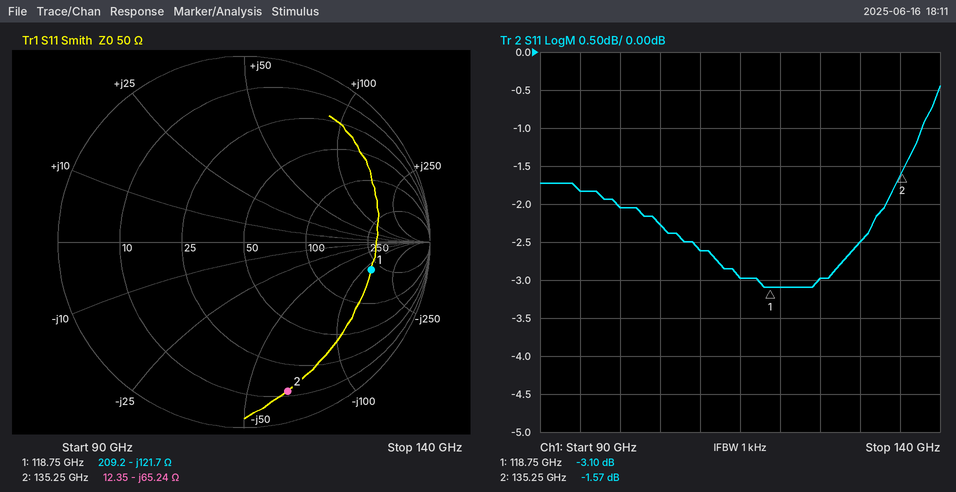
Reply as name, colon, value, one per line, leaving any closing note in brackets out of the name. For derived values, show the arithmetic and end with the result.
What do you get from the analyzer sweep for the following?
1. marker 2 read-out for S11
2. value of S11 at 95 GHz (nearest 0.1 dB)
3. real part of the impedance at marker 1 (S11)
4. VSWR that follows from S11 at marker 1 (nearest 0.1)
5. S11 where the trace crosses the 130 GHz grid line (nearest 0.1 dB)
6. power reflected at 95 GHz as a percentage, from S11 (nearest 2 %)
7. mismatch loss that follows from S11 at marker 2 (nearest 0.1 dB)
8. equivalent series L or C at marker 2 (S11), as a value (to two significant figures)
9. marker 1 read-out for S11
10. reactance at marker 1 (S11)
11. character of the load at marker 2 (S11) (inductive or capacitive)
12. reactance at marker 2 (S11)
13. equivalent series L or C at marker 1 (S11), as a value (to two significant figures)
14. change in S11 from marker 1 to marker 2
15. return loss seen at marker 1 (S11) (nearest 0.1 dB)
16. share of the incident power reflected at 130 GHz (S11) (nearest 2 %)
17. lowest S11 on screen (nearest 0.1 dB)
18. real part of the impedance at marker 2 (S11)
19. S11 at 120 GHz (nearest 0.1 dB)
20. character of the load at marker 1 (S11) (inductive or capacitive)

marker 2 read-out for S11: -1.57 dB
value of S11 at 95 GHz: -1.8 dB
real part of the impedance at marker 1: 209.2 Ω
VSWR that follows from S11 at marker 1: (1 + 0.6998)/(1 − 0.6998) ≈ 5.7
S11 where the trace crosses the 130 GHz grid line: -2.5 dB
power reflected at 95 GHz as a percentage, from S11: 10^(-1.8/10) ≈ 66 %
mismatch loss that follows from S11 at marker 2: −10 log10(1 − 10^(-1.57/10)) ≈ 5.2 dB
equivalent series L or C at marker 2 (S11), as a value: C = 1/(2π × 135.25 GHz × 65.24 Ω) ≈ 18 fF
marker 1 read-out for S11: -3.10 dB
reactance at marker 1: -121.7 Ω
character of the load at marker 2 (S11): capacitive
reactance at marker 2: -65.24 Ω
equivalent series L or C at marker 1 (S11), as a value: C = 1/(2π × 118.75 GHz × 121.7 Ω) ≈ 11 fF
change in S11 from marker 1 to marker 2: -1.57 − (-3.1) = 1.53 dB
return loss seen at marker 1 (S11): 3.1 dB
share of the incident power reflected at 130 GHz (S11): 10^(-2.5/10) ≈ 56 %
lowest S11 on screen: -3.1 dB
real part of the impedance at marker 2: 12.35 Ω
S11 at 120 GHz: -3.1 dB
character of the load at marker 1 (S11): capacitive
